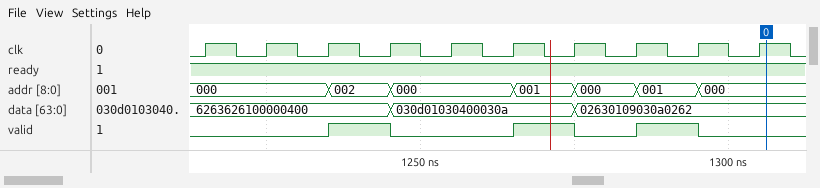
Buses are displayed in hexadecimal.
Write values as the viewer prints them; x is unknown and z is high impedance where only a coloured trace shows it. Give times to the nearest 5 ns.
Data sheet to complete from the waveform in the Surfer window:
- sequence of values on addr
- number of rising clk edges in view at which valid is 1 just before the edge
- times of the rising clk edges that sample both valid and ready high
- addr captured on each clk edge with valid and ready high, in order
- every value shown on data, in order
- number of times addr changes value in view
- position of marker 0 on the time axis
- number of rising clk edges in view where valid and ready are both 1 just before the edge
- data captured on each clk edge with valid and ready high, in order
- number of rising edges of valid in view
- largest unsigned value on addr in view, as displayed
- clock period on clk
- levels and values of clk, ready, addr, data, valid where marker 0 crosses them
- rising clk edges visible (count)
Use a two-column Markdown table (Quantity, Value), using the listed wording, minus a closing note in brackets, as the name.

| Quantity | Value |
|---|---|
| sequence of values on addr | 000, 002, 000, 001, 000, 001, 000 |
| number of rising clk edges in view at which valid is 1 just before the edge | 3 |
| times of the rising clk edges that sample both valid and ready high | 1245 ns, 1275 ns, 1295 ns |
| addr captured on each clk edge with valid and ready high, in order | 002, 001, 001 |
| every value shown on data, in order | 6263626100000400, 030d01030400030a, 02630109030a0262 |
| number of times addr changes value in view | 6 |
| position of marker 0 on the time axis | 1305 ns |
| number of rising clk edges in view where valid and ready are both 1 just before the edge | 3 |
| data captured on each clk edge with valid and ready high, in order | 6263626100000400, 030d01030400030a, 02630109030a0262 |
| number of rising edges of valid in view | 3 |
| largest unsigned value on addr in view, as displayed | 002 |
| clock period on clk | 10 ns |
| levels and values of clk, ready, addr, data, valid where marker 0 crosses them | clk=1, ready=1, addr=000, data=02630109030a0262, valid=0 |
| rising clk edges visible | 10 |
